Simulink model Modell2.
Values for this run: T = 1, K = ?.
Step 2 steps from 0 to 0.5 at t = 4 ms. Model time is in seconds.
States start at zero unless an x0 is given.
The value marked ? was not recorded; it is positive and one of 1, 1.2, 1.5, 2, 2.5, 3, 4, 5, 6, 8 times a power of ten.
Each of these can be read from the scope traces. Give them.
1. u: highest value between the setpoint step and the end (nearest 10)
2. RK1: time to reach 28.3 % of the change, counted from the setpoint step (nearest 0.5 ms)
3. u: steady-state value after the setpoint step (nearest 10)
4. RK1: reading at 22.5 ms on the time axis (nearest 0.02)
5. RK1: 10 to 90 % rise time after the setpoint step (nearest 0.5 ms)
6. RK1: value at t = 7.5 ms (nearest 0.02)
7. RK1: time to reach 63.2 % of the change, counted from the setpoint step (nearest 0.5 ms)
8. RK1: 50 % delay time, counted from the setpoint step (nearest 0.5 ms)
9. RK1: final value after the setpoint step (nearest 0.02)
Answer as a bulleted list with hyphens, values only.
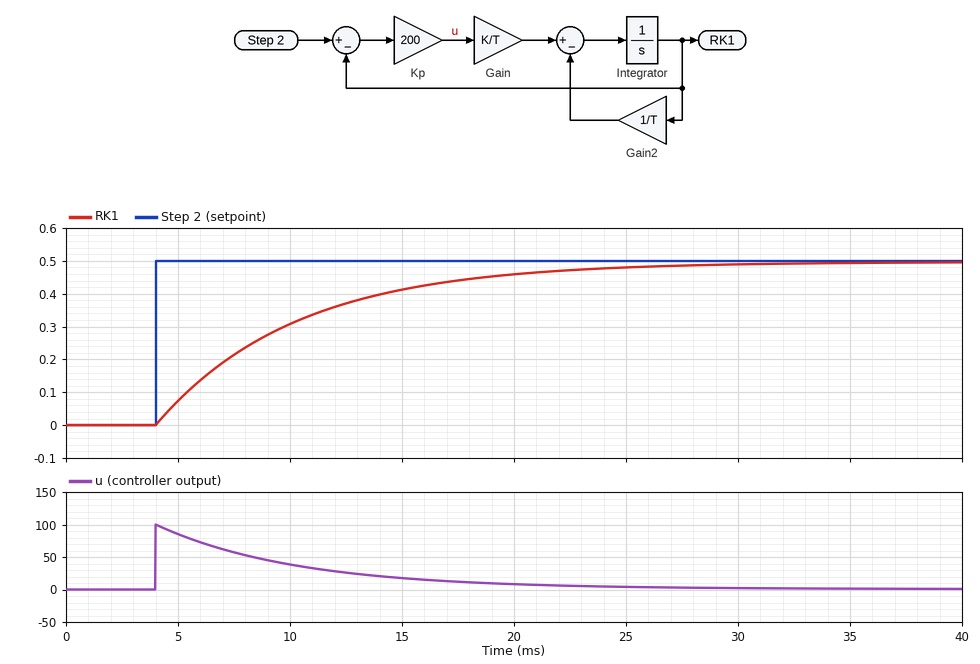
- 100
- 2.0 ms
- 0
- 0.48
- 13.5 ms
- 0.22
- 6.0 ms
- 4.5 ms
- 0.50
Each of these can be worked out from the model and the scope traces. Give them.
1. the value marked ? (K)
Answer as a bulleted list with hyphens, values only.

- 0.8
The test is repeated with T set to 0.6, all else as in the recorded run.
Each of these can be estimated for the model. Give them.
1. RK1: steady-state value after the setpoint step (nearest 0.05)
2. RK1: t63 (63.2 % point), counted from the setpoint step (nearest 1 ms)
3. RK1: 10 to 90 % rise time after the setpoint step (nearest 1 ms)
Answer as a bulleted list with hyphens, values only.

- 0.50
- 4 ms
- 8 ms
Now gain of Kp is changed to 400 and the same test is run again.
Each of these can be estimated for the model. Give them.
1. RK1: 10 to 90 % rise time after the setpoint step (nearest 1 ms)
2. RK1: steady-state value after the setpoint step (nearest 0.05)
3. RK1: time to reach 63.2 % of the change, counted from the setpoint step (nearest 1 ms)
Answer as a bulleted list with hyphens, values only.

- 7 ms
- 0.50
- 3 ms
